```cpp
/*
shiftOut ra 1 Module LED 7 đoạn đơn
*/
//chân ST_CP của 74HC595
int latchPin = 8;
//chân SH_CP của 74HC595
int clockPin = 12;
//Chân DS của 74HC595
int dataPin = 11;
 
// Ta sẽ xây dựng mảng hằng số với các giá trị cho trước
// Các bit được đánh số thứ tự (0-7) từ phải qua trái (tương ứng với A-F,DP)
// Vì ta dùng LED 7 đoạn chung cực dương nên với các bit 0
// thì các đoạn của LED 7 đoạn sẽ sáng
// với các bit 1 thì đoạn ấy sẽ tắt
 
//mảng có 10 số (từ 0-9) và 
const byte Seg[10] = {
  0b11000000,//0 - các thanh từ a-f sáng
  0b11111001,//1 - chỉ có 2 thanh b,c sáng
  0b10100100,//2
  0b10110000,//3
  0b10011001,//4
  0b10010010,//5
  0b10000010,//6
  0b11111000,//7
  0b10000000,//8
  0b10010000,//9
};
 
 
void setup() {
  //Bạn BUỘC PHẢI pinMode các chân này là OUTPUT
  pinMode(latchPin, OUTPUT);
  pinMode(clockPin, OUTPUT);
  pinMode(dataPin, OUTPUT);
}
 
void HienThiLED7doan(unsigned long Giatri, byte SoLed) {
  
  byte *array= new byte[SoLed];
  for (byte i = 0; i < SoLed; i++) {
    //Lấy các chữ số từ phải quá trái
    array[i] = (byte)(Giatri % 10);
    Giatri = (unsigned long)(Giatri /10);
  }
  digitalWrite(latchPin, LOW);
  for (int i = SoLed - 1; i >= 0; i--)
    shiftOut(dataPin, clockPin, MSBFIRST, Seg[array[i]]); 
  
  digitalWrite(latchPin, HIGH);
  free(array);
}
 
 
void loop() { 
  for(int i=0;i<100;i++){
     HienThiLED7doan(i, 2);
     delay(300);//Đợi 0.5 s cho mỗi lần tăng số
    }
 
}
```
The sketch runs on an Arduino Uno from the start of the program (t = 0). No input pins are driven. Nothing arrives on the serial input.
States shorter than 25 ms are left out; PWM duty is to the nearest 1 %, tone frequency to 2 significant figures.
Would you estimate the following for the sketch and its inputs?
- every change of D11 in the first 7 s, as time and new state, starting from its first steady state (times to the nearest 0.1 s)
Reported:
0 s low; 0.3 s high; 0.6 s low; 1.2 s high; 1.5 s low; 3.3 s high; 3.6 s low; 4.2 s high; 4.5 s low; 6.3 s high; 6.6 s low
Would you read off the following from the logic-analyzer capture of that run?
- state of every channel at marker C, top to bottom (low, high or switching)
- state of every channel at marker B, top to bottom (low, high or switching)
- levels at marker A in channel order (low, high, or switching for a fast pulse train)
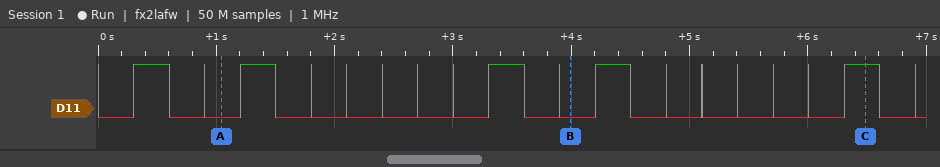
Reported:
D11 high
D11 low
D11 low
